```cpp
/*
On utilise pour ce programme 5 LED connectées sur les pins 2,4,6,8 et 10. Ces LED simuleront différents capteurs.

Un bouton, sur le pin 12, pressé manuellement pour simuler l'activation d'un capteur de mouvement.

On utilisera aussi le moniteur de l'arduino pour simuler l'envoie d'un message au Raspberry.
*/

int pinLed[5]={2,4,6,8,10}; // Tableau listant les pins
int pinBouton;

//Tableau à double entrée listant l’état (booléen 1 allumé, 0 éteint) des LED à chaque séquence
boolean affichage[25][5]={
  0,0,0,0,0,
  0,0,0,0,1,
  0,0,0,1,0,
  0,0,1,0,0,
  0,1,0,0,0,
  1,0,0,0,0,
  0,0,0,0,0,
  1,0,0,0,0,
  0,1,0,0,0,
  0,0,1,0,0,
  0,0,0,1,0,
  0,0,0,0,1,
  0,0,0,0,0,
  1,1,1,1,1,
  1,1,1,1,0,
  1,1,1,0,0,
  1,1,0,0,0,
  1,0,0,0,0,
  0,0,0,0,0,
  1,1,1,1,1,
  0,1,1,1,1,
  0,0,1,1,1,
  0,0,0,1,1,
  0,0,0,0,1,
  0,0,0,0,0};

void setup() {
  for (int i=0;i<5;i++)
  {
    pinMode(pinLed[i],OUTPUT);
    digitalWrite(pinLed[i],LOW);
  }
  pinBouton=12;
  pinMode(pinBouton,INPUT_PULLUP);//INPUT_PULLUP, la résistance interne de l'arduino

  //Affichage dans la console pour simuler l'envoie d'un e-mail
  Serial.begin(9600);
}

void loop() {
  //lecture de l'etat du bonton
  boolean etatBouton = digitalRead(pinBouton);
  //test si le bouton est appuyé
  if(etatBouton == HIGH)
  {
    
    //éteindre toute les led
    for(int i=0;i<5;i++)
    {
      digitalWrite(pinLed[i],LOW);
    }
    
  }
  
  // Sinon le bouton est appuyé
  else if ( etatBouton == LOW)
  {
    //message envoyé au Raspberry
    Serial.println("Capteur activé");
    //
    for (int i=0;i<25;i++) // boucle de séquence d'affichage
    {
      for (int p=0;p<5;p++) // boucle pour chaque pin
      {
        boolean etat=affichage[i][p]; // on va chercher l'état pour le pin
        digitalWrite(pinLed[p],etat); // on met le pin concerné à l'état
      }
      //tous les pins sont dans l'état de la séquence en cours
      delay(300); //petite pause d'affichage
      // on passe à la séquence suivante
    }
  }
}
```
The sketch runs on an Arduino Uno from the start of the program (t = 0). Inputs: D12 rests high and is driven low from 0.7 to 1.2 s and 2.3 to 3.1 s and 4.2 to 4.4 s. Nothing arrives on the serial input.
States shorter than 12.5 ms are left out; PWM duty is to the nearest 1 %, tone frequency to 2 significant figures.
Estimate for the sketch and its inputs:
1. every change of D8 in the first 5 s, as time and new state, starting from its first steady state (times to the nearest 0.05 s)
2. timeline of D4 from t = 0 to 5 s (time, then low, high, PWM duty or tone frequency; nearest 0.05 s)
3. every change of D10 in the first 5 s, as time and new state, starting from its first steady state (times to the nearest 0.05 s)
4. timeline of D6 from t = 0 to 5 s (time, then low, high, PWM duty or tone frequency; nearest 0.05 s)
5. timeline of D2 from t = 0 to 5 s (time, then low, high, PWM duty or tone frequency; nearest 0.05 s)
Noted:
0 s low; 1.3 s high; 1.6 s low; 3.7 s high; 4 s low; 4.6 s high
0 s low; 1.9 s high; 2.2 s low; 3.1 s high; 3.4 s low; 4.6 s high
0 s low; 1 s high; 1.3 s low; 4 s high; 4.3 s low; 4.6 s high; 4.9 s low
0 s low; 1.6 s high; 1.9 s low; 3.4 s high; 3.7 s low; 4.6 s high
0 s low; 2.2 s high; 2.5 s low; 2.8 s high; 3.1 s low; 4.6 s high
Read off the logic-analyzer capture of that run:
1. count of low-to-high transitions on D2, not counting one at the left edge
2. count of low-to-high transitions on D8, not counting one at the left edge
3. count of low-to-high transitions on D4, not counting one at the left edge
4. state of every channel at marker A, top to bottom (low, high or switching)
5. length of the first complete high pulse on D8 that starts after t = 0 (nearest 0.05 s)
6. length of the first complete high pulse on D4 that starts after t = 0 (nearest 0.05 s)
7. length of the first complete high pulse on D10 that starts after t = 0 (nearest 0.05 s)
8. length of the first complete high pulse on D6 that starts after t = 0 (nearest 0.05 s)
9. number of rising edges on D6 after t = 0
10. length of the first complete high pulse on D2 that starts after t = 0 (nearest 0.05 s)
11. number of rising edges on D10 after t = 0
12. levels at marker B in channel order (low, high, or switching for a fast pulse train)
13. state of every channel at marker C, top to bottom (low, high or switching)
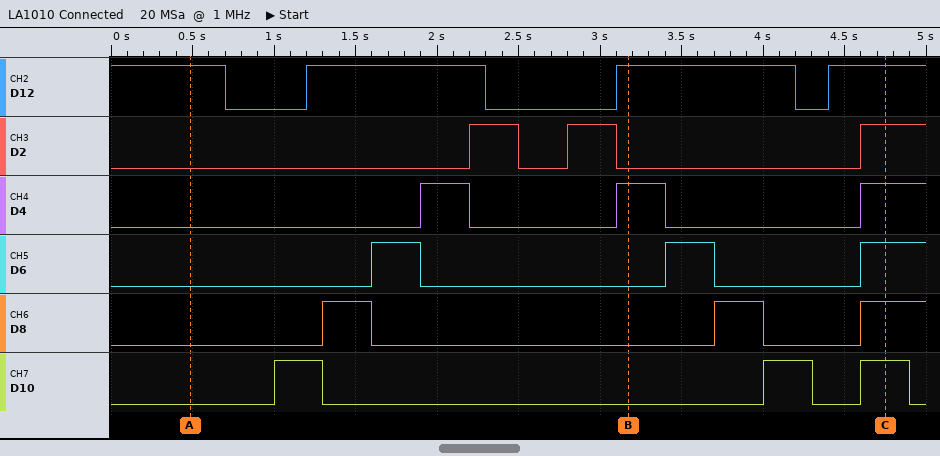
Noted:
3
3
3
D12 high, D2 low, D4 low, D6 low, D8 low, D10 low
0.30 s
0.30 s
0.30 s
0.30 s
3
0.30 s
3
D12 high, D2 low, D4 high, D6 low, D8 low, D10 low
D12 high, D2 high, D4 high, D6 high, D8 high, D10 high
